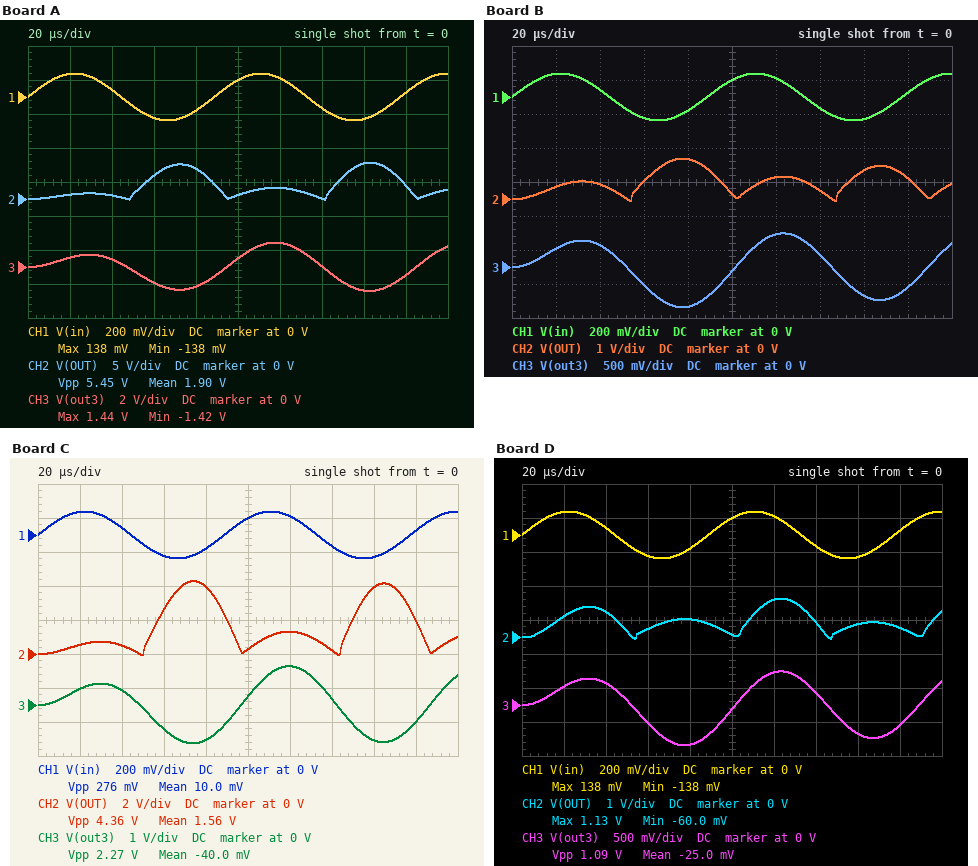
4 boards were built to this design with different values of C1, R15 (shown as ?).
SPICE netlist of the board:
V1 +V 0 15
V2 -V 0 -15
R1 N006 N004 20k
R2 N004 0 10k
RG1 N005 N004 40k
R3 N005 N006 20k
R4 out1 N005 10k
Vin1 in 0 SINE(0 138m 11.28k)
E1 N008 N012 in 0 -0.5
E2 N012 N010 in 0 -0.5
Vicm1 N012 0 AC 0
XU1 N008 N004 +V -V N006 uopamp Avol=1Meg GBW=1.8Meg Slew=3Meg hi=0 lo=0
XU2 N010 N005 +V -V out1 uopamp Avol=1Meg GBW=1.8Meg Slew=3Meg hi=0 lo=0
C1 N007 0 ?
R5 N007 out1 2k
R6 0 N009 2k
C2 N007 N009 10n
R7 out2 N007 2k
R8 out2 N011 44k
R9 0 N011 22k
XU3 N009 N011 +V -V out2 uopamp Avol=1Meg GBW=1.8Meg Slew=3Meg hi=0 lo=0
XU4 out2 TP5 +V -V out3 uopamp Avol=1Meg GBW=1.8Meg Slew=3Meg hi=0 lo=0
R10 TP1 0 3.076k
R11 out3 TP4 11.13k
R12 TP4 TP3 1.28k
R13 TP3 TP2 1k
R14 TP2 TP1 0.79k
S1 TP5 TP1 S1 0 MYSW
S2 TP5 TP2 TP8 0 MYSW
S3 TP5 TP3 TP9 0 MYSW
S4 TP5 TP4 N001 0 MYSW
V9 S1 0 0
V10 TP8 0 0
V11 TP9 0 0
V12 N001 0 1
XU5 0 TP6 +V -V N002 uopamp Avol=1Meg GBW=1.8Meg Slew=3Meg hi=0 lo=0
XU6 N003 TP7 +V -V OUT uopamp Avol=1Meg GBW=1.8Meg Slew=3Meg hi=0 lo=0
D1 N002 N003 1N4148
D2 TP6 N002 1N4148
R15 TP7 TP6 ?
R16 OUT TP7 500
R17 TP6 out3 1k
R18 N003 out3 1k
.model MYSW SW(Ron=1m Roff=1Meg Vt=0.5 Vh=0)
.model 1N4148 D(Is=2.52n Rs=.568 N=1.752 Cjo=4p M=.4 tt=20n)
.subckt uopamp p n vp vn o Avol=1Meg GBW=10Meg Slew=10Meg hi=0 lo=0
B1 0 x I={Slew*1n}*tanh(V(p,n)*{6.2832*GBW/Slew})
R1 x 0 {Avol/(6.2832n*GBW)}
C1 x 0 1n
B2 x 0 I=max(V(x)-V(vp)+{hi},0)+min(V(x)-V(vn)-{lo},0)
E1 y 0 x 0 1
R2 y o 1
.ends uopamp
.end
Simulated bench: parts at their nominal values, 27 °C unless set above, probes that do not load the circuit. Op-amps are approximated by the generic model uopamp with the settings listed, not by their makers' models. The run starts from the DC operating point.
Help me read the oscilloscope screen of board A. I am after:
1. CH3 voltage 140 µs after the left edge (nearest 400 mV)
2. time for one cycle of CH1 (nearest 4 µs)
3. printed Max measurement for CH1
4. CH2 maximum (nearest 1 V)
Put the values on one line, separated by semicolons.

0 V; 88 µs; 138 mV; 5 V
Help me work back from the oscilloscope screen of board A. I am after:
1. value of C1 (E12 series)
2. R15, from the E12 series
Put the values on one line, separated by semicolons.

15 nF; 3.3 kΩ
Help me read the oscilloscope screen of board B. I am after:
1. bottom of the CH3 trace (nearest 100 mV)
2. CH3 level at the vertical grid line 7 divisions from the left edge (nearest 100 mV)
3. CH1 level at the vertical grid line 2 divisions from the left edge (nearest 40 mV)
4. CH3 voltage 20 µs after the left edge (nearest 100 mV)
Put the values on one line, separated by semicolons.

-600 mV; 200 mV; 40 mV; 300 mV
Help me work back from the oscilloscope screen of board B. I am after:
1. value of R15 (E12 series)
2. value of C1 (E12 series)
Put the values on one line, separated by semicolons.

1.5 kΩ; 33 nF
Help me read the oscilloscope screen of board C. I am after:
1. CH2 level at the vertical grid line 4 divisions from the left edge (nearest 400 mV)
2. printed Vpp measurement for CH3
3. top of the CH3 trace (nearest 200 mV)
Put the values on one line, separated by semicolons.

4.0 V; 2.27 V; 1.2 V
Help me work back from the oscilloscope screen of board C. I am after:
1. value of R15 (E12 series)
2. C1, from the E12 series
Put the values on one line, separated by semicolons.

3.3 kΩ; 18 nF
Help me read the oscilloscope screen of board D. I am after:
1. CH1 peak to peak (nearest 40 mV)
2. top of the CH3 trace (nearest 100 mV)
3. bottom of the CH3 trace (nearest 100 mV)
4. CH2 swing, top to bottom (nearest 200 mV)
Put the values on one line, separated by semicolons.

280 mV; 500 mV; -600 mV; 1.2 V
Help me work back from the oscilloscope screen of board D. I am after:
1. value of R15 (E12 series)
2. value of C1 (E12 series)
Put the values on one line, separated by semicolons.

390 Ω; 33 nF
